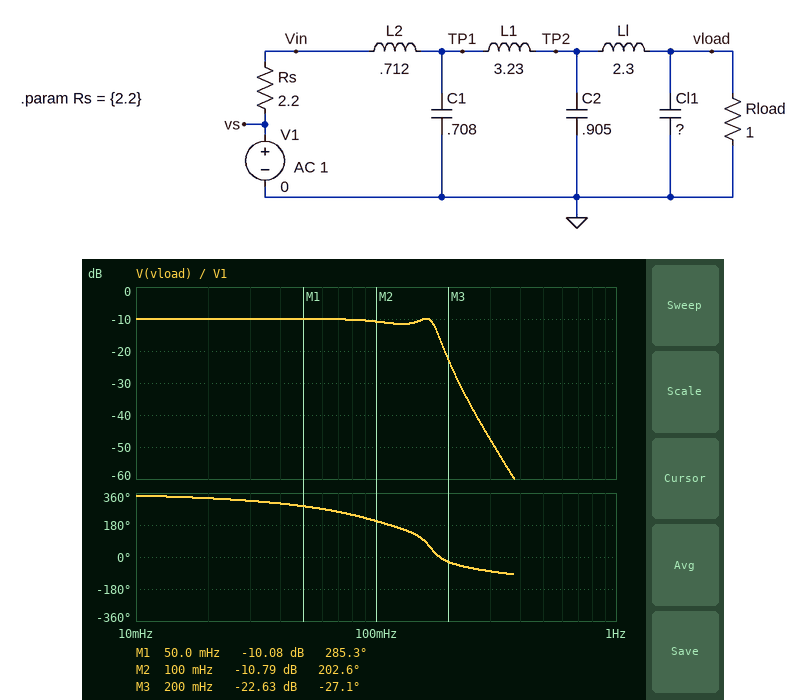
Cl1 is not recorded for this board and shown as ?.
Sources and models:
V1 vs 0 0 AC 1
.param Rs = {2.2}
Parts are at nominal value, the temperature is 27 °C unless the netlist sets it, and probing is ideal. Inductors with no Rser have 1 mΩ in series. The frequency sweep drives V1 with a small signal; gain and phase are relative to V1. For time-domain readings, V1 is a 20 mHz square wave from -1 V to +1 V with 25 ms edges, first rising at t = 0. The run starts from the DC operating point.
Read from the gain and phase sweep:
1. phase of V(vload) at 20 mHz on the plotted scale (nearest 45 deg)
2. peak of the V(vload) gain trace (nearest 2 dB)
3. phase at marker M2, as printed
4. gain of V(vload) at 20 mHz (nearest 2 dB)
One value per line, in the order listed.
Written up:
315 deg
-10 dB
202.6 deg
-10 dB
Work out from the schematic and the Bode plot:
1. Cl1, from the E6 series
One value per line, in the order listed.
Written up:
1.5 F
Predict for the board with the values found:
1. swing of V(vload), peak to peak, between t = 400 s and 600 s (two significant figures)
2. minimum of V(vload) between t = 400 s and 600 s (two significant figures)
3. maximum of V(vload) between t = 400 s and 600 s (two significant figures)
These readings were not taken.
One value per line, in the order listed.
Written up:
800 mV
-400 mV
400 mV
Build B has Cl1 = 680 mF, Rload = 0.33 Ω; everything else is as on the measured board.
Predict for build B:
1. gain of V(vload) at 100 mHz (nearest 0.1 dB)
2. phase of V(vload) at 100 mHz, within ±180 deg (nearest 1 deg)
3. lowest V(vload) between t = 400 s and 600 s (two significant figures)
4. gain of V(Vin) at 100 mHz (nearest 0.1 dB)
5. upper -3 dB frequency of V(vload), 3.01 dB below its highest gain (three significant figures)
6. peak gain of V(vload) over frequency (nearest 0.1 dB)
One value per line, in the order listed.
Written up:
-17.3 dB
-135 deg
-190 mV
-3.8 dB
172 mHz
-15.4 dB
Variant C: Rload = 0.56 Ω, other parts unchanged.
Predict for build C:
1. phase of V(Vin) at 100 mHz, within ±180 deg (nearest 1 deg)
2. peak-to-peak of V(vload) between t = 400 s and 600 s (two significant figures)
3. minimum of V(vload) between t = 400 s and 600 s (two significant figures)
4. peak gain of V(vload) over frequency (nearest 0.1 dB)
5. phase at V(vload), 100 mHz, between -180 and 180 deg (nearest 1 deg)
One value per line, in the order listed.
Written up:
-26 deg
560 mV
-280 mV
-12.6 dB
-149 deg
